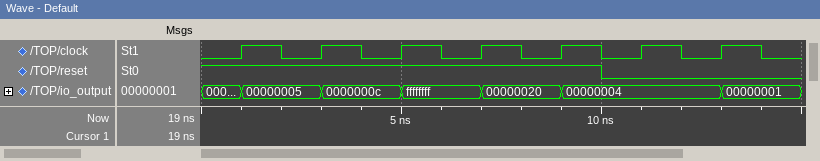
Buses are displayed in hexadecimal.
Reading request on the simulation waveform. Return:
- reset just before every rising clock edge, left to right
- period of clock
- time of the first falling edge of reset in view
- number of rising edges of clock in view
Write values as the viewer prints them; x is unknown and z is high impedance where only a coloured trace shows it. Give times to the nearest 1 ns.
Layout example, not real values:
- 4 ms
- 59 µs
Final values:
- 1 1 1 1 1 0 0
- 2 ns
- 10 ns
- 7
